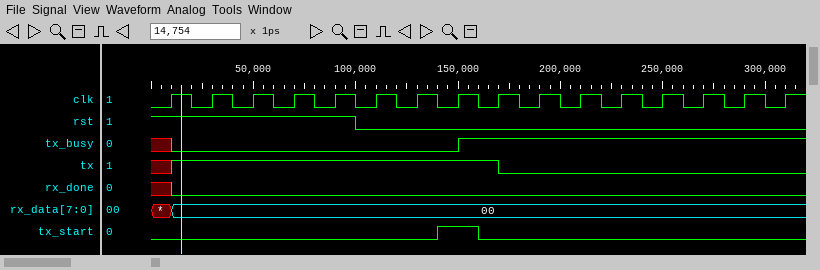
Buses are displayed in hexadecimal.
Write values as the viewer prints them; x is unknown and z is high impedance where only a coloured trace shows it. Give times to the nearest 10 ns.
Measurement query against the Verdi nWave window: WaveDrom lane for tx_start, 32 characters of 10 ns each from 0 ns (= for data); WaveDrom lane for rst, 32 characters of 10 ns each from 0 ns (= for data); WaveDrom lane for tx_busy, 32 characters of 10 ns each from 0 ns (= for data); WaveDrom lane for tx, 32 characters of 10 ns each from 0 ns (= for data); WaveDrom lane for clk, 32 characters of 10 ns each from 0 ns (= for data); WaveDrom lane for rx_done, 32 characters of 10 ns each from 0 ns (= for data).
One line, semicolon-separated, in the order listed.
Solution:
{name: 'tx_start', wave: '0.............1.0...............'}; {name: 'rst', wave: '1.........0.....................'}; {name: 'tx_busy', wave: 'x0.............1................'}; {name: 'tx', wave: 'x1...............0..............'}; {name: 'clk', wave: '01010101010101010101010101010101'}; {name: 'rx_done', wave: 'x0..............................'}
